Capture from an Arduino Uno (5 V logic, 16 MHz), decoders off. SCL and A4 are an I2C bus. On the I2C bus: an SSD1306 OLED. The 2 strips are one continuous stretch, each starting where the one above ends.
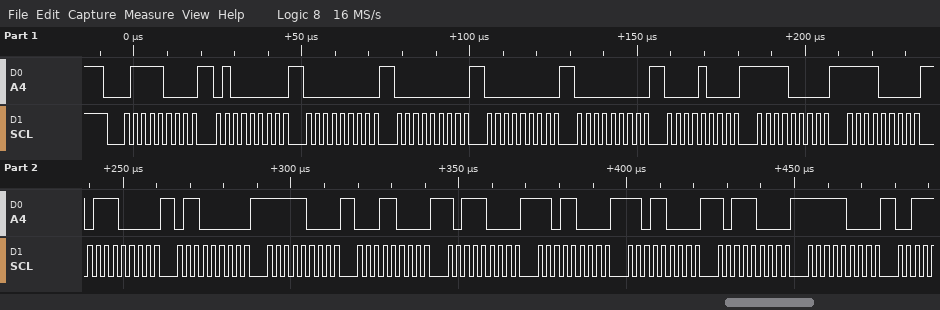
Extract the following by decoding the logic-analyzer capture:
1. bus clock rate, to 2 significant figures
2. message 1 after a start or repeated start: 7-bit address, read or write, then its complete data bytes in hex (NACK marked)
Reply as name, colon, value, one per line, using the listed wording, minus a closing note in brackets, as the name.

bus clock rate, to 2 significant figures: 400 kHz
message 1 after a start or repeated start: 7-bit address, read or write, then its complete data bytes in hex: 0x3C write: 40 00 00 00 00 08 F0 F0 70 60 F8 18 B8 D8 D8 B8 F8
